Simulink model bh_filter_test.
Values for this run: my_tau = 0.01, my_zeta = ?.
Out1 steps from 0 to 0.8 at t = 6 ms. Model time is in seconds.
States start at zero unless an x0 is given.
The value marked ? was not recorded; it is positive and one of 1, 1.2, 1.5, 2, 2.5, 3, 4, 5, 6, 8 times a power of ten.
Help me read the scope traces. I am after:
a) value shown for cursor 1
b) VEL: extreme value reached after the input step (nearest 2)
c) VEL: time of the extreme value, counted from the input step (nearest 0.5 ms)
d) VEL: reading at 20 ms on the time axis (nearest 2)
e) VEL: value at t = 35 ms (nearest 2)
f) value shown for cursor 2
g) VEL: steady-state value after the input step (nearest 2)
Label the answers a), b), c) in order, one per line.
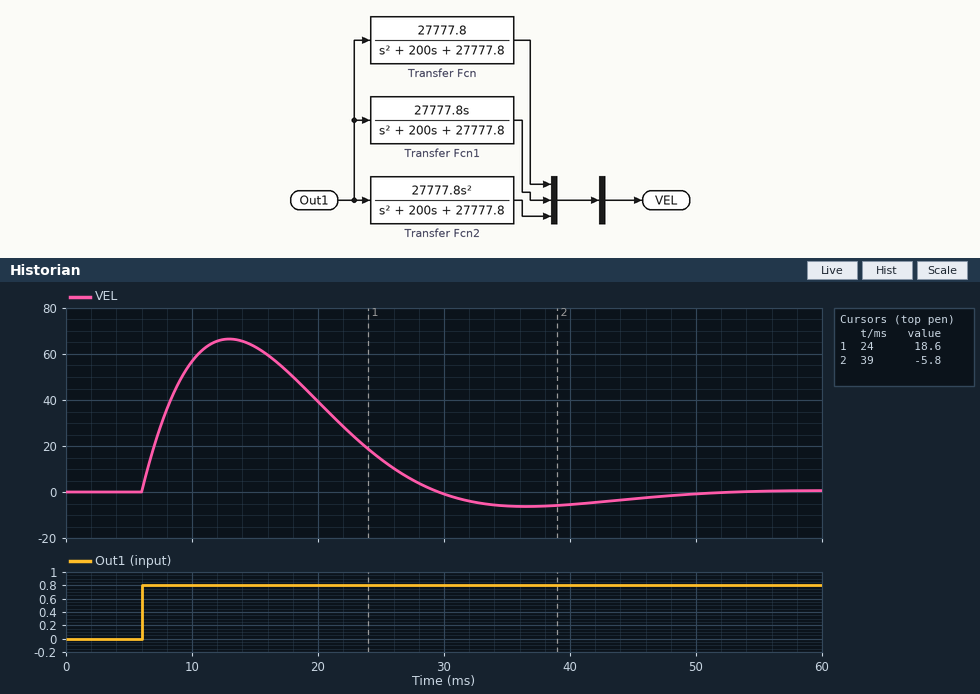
a) 18.6
b) 66
c) 7.0 ms
d) 40
e) -6
f) -5.8
g) 0
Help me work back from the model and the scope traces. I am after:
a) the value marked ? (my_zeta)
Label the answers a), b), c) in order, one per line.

a) 0.6
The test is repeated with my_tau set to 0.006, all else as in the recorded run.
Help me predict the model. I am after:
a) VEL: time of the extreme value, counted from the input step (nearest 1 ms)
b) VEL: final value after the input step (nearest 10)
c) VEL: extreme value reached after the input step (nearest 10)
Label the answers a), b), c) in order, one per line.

a) 4 ms
b) 0
c) 110
